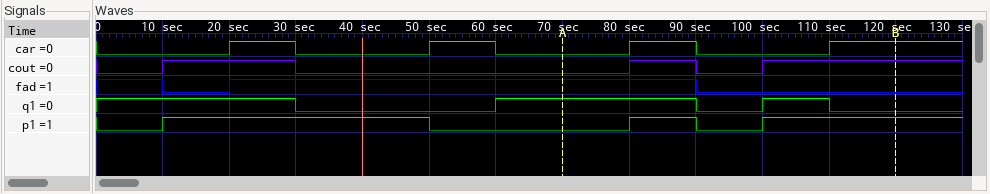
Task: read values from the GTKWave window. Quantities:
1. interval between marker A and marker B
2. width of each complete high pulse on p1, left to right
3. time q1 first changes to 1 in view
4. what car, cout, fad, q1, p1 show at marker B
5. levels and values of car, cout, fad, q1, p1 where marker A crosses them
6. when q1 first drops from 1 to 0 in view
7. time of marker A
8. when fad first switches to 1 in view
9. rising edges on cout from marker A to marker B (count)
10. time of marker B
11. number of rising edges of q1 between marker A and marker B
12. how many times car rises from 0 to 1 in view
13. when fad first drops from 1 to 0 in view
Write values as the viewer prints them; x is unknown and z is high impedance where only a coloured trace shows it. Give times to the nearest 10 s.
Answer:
50 s
40 s, 10 s
60 s
car=1, cout=1, fad=0, q1=0, p1=1
car=0, cout=0, fad=1, q1=1, p1=0
30 s
70 s
20 s
2
120 s
1
4
10 s
